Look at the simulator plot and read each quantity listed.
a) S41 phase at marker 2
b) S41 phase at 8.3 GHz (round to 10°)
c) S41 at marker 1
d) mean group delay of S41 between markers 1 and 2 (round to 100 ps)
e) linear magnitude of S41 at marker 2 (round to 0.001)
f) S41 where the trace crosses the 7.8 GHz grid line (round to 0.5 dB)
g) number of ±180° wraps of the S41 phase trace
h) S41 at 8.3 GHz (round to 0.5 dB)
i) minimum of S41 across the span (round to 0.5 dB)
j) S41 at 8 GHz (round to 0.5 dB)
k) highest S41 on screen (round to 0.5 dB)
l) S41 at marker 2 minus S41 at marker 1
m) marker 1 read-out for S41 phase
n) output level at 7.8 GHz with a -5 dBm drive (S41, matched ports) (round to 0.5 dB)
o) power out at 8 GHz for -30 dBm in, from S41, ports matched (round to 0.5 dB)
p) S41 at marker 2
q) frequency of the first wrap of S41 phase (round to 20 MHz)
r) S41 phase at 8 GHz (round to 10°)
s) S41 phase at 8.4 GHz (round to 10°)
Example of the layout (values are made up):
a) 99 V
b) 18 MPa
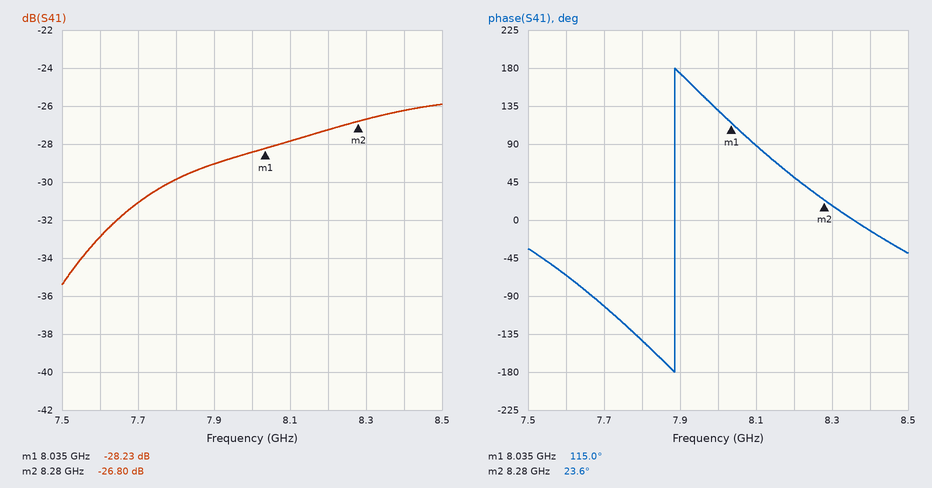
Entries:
a) 23.6°
b) 20°
c) -28.23 dB
d) 1.0 ns
e) 0.046
f) -30.0 dB
g) 1
h) -26.5 dB
i) -35.5 dB
j) -28.5 dB
k) -26.0 dB
l) 1.43 dB
m) 115.0°
n) -35.0 dBm
o) -58.5 dBm
p) -26.80 dB
q) 7.88 GHz
r) 130°
s) -10°
